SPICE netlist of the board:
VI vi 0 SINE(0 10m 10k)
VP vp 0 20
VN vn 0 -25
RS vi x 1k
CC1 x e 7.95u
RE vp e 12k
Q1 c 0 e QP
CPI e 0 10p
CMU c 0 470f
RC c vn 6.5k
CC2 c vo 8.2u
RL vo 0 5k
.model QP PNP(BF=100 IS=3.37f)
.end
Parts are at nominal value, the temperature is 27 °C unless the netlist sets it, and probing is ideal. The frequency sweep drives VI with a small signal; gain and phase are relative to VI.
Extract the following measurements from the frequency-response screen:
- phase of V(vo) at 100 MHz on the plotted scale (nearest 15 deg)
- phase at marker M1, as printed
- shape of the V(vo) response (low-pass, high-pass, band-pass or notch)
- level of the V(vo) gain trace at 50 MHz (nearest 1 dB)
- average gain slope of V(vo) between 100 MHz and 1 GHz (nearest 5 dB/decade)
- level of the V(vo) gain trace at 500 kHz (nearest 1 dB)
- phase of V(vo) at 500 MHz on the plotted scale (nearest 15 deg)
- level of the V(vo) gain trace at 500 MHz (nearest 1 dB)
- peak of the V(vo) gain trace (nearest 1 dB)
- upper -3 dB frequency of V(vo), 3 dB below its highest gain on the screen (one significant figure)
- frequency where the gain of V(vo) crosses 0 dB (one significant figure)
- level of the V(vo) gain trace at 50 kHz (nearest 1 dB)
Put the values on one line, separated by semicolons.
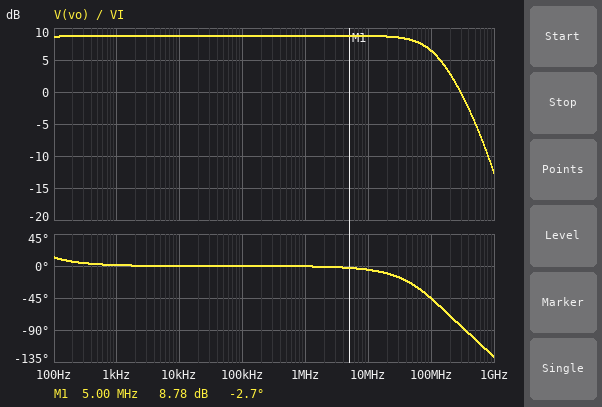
-45 deg; -2.7 deg; low-pass; 8 dB; -20 dB/decade; 9 dB; -105 deg; -5 dB; 9 dB; 100 MHz; 300 MHz; 9 dB
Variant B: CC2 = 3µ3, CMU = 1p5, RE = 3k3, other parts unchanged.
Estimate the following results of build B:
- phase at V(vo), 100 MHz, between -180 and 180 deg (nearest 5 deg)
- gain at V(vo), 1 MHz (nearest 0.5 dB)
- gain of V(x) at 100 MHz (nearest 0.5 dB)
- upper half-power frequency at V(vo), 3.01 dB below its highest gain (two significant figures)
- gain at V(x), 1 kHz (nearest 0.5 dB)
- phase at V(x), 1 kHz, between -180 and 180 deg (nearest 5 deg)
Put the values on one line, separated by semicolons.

-5 deg; -37.0 dB; -43.5 dB; 2.0 GHz; -33.5 dB; -70 deg
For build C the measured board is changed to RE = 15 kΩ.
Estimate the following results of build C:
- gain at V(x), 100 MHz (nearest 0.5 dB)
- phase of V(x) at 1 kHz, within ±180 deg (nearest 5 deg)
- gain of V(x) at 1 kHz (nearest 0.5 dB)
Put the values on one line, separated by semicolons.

-34.0 dB; -45 deg; -31.0 dB
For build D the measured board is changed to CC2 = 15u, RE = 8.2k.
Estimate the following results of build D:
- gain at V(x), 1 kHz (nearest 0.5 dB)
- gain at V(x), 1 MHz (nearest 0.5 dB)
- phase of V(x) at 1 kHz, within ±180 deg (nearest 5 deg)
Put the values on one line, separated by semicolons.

-33.0 dB; -39.5 dB; -60 deg
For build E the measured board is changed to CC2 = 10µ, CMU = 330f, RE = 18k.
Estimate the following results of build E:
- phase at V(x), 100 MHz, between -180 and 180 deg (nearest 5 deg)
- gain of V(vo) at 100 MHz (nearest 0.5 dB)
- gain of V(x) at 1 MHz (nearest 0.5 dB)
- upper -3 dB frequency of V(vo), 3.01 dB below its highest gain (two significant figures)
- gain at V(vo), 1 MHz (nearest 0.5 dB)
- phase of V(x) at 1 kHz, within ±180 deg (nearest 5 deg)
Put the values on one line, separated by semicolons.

-10 deg; 7.5 dB; -32.5 dB; 160 MHz; 8.5 dB; -40 deg
